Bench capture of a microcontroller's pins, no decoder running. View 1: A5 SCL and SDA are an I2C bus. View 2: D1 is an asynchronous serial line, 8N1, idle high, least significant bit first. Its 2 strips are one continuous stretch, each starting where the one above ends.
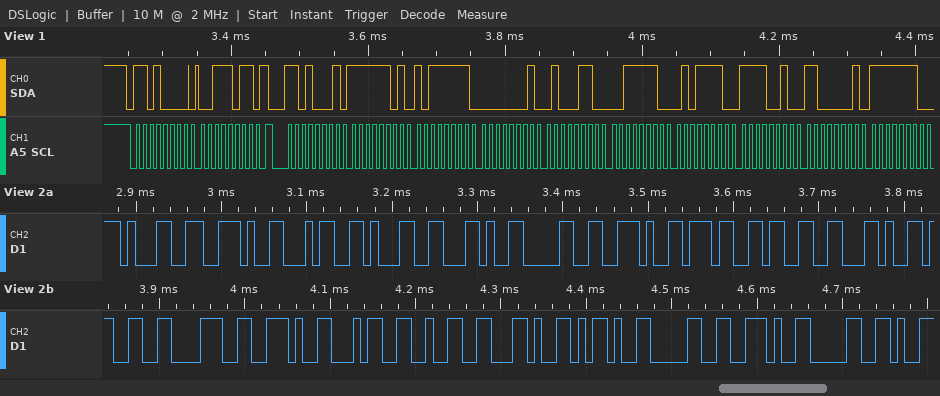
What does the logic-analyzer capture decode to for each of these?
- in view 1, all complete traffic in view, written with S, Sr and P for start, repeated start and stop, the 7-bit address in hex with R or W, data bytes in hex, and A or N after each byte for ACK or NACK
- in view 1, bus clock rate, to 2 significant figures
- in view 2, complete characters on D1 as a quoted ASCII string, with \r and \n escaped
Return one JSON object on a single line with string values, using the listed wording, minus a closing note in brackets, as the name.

{"in view 1, all complete traffic in view, written with S, Sr and P for start, repeated start and stop, the 7-bit address in hex with R or W, data bytes in hex, and A or N after each byte for ACK or NACK": "S 68W A 3B A Sr 68R A FD A BF A 01 A 46 A 3E A 5E A F2 A C1 A FE A", "in view 1, bus clock rate, to 2 significant figures": "100 kHz", "in view 2, complete characters on D1 as a quoted ASCII string, with \\r and \\n escaped": "\"1.41,0.73,38.42,-0.0\""}
